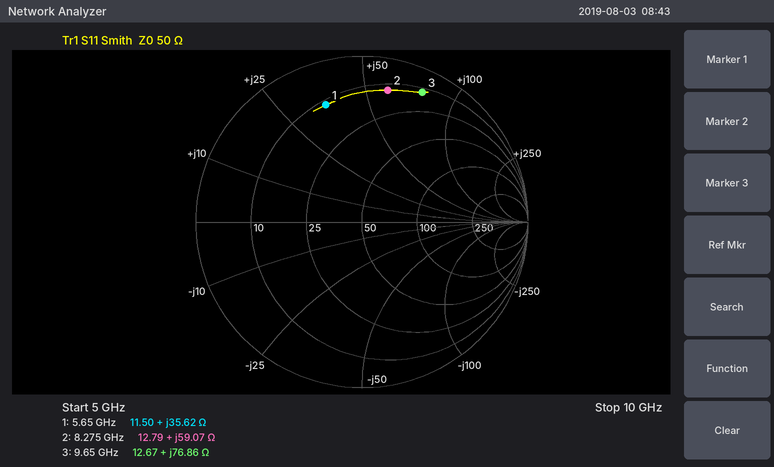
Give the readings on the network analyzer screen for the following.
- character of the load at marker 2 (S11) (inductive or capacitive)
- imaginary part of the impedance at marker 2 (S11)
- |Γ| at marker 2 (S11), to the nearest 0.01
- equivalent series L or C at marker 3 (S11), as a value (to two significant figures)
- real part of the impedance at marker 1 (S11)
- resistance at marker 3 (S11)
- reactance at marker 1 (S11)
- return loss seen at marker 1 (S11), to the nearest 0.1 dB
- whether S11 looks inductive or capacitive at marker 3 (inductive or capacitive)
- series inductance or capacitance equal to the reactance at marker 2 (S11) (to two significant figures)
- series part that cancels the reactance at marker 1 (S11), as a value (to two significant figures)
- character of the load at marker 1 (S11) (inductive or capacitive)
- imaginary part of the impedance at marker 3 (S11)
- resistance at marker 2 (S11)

inductive
+59.07 Ω
0.81
1.3 nH
11.50 Ω
12.67 Ω
+35.62 Ω
2.6 dB
inductive
1.1 nH
790 fF
inductive
+76.86 Ω
12.79 Ω
